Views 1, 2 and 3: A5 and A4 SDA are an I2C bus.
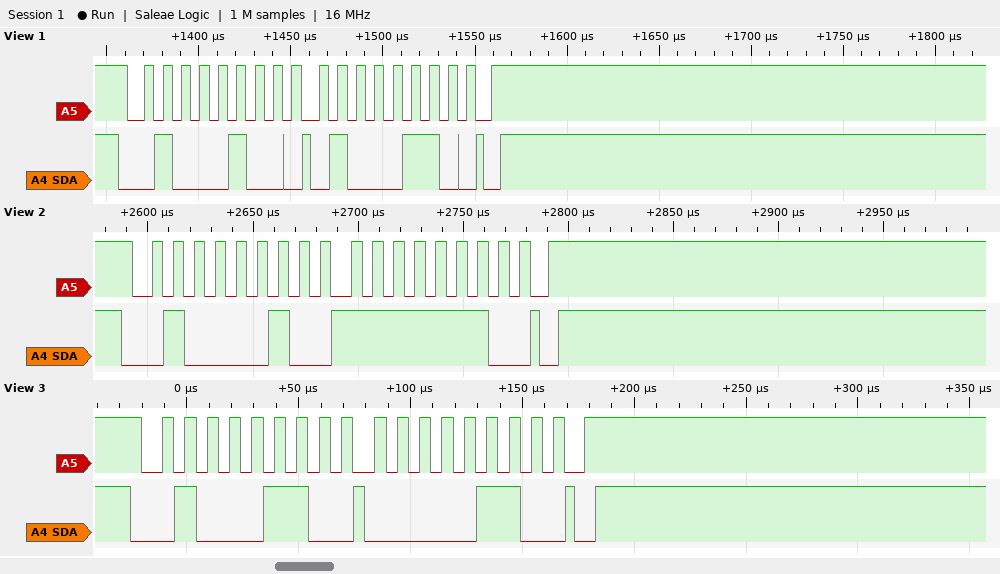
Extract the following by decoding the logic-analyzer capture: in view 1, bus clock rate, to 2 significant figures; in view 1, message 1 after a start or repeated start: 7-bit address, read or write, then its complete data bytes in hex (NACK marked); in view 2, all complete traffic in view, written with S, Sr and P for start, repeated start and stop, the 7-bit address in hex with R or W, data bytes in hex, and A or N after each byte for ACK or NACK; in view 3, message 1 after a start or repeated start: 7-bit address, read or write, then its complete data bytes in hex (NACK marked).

100 kHz
0x22 write: 46
S 21W A FE A P
0x23 write: 06
